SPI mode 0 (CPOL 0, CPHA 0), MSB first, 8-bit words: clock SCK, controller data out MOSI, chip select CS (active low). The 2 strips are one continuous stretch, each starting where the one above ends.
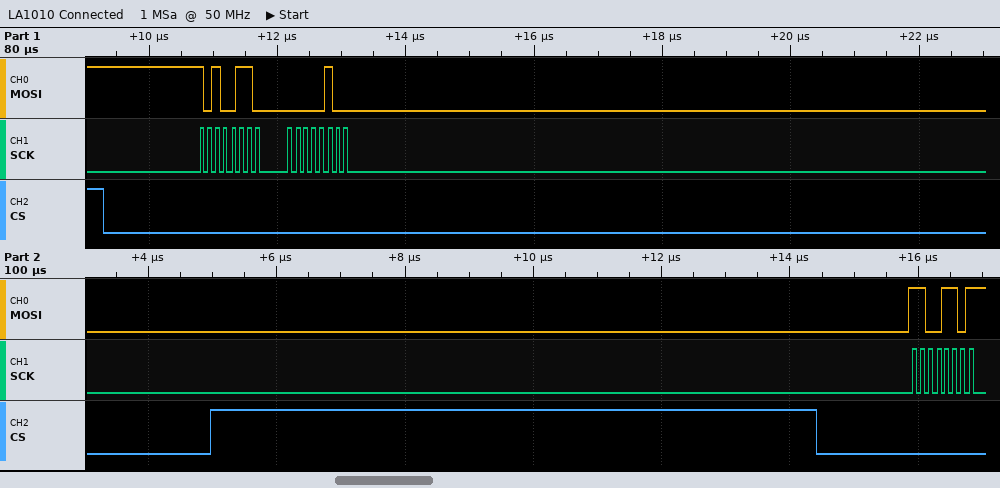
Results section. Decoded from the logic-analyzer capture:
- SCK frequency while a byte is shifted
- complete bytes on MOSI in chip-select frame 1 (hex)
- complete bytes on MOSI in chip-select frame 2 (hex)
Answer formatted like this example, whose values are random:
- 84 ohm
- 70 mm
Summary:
- 8 MHz
- A6 04
- CD
